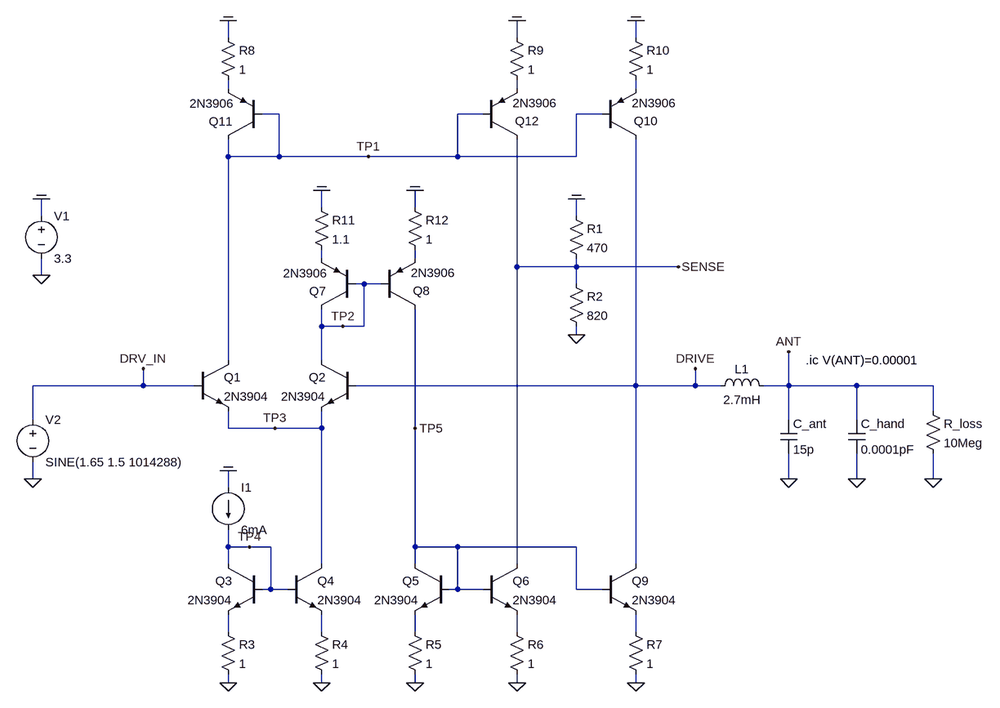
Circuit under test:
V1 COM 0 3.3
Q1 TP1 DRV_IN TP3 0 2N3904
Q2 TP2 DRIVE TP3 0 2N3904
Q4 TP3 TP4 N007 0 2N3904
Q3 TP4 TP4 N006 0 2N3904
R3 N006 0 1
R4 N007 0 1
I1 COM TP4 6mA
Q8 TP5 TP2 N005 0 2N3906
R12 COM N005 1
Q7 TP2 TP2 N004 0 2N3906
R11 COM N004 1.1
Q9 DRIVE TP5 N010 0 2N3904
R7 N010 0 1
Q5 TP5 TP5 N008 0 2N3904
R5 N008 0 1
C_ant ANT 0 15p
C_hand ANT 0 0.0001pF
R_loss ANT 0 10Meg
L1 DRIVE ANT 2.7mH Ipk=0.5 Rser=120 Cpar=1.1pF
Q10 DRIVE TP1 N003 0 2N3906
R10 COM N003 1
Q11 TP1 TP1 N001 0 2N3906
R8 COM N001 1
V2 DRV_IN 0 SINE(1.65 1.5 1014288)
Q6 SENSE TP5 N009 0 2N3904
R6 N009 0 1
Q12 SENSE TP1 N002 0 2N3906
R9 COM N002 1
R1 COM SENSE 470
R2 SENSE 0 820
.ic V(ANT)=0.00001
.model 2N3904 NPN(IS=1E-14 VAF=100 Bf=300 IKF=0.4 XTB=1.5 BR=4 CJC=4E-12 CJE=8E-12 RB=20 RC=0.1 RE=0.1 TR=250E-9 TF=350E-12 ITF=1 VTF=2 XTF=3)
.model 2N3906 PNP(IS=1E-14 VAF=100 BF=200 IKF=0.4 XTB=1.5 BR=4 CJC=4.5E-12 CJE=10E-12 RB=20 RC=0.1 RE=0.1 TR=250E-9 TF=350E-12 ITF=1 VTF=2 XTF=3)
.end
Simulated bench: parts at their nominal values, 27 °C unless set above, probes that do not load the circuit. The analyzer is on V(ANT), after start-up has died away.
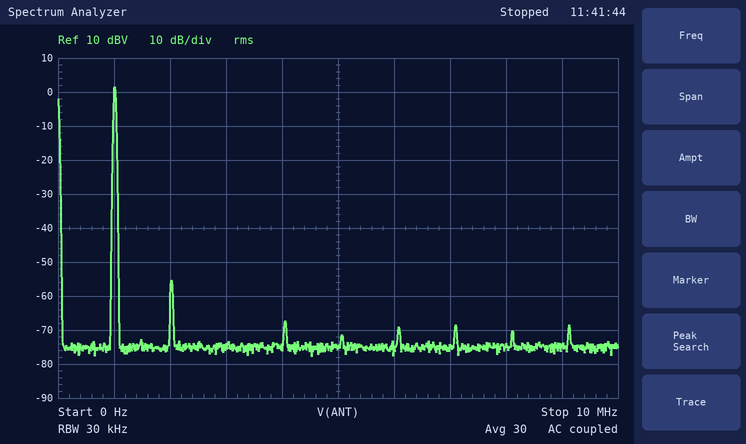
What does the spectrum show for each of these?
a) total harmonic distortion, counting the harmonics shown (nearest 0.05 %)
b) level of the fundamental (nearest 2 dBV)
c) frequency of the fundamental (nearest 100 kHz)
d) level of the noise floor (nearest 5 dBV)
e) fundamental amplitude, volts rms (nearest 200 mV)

0.15 %
2 dBV
1.0 MHz
-75 dBV
1.2 V
